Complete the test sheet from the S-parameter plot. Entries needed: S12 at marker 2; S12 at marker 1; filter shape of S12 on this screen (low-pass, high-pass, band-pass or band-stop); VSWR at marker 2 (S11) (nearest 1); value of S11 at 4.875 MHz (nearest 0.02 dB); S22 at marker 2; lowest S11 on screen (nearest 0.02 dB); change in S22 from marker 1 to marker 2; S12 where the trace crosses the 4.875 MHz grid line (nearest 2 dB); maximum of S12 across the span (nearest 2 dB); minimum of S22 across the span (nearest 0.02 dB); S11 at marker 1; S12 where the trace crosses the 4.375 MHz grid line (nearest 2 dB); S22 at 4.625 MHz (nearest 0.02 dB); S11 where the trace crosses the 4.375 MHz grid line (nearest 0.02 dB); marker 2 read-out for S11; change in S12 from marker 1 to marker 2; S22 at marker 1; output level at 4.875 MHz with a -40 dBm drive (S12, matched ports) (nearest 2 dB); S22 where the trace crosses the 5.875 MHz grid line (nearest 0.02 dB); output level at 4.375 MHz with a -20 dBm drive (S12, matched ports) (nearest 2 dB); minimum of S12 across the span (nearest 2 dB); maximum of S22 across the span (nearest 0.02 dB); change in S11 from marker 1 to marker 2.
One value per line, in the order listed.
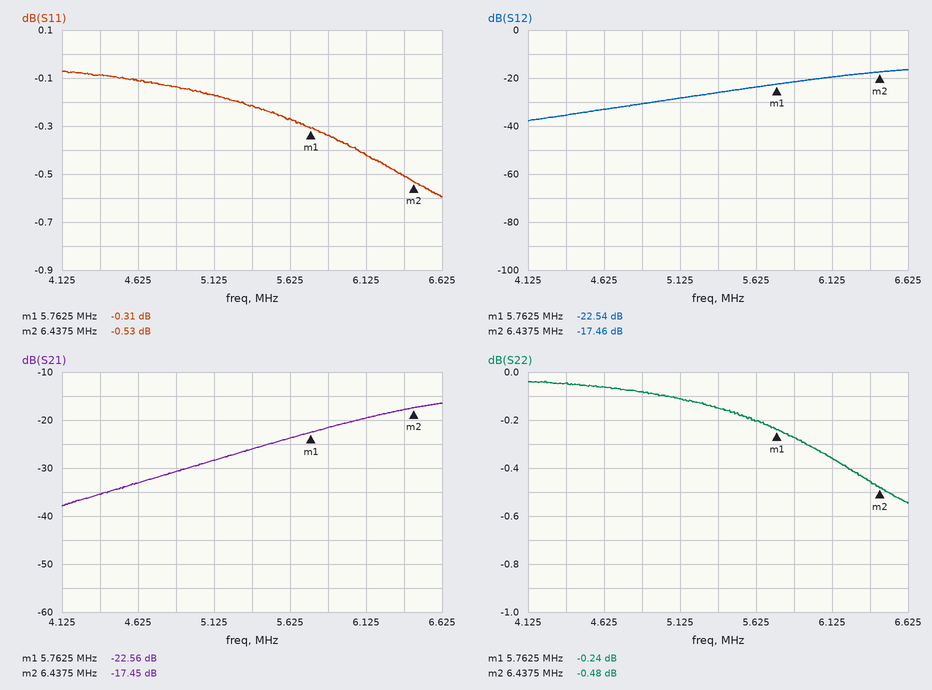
-17.46 dB
-22.54 dB
high-pass
33
-0.14 dB
-0.48 dB
-0.60 dB
-0.24 dB
-30 dB
-16 dB
-0.54 dB
-0.31 dB
-36 dB
-0.06 dB
-0.08 dB
-0.53 dB
5.08 dB
-0.24 dB
-70 dBm
-0.28 dB
-56 dBm
-38 dB
-0.04 dB
-0.22 dB
